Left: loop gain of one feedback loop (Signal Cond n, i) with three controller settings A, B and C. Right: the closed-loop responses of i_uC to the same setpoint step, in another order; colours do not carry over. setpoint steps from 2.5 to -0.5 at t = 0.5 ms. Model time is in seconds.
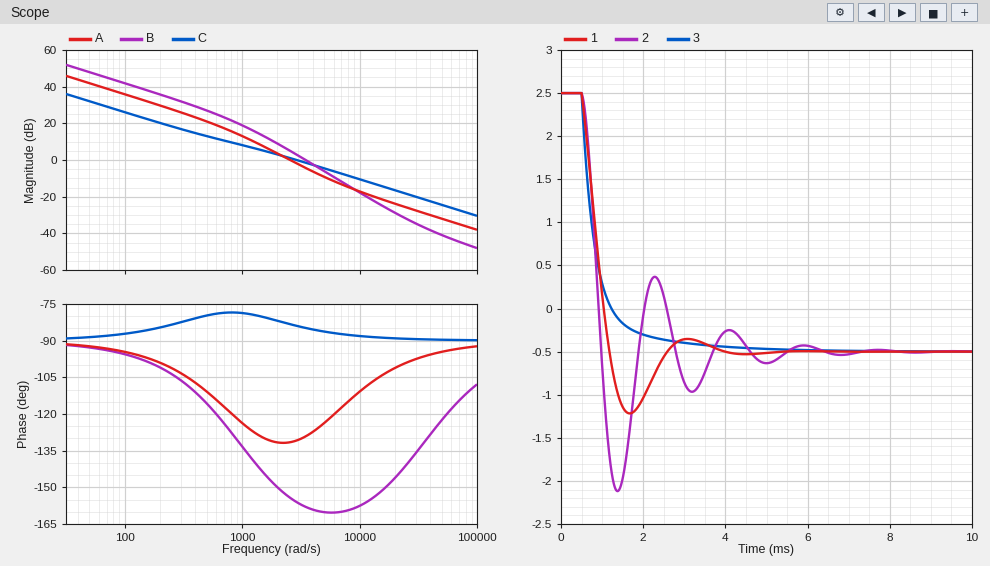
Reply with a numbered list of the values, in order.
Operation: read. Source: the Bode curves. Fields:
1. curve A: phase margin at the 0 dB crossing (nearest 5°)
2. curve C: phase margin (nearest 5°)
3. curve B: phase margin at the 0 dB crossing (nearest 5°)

1. 50°
2. 95°
3. 20°
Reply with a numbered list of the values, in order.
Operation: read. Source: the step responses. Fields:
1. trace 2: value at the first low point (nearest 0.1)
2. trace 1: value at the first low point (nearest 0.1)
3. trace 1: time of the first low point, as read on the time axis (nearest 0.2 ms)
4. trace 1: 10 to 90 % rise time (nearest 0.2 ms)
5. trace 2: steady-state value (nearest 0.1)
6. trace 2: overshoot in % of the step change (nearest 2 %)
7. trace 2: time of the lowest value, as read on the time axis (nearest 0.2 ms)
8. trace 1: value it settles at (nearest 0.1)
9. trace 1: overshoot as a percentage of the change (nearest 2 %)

1. -2.1
2. -1.2
3. 1.6 ms
4. 0.6 ms
5. -0.5
6. 54 %
7. 1.4 ms
8. -0.5
9. 24 %
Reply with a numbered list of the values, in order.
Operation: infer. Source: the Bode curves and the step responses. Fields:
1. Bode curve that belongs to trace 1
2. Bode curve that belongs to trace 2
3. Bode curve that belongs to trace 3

1. A
2. B
3. C
